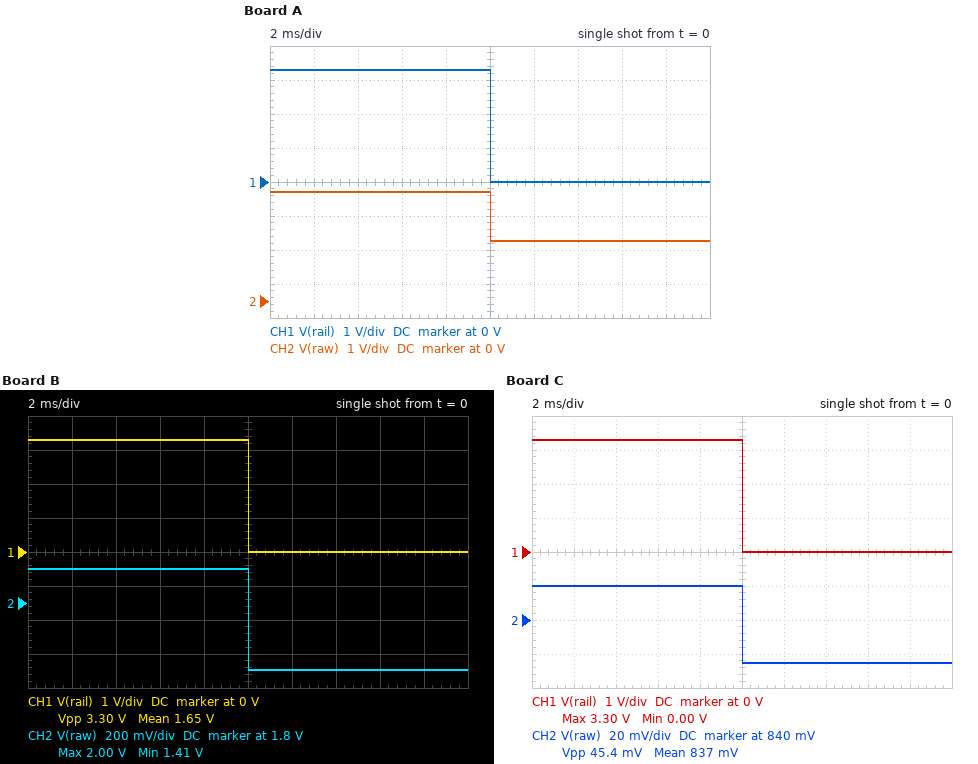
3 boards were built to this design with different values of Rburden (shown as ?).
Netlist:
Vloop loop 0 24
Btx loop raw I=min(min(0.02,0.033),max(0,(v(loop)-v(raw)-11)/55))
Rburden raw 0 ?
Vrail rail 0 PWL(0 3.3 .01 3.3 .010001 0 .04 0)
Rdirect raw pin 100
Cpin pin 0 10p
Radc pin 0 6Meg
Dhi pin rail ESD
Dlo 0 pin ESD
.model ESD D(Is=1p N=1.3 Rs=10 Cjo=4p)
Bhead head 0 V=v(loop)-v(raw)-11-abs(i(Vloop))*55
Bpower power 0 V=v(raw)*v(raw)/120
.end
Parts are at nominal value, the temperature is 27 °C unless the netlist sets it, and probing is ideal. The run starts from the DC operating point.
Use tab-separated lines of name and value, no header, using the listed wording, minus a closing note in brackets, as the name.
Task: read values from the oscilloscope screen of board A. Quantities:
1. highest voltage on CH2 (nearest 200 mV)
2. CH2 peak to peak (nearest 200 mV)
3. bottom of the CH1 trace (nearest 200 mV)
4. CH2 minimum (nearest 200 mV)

highest voltage on CH2	3.2 V
CH2 peak to peak	1.4 V
bottom of the CH1 trace	0 V
CH2 minimum	1.8 V
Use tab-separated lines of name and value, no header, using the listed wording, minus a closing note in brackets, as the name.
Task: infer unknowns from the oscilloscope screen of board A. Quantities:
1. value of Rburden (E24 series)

value of Rburden	160 Ω
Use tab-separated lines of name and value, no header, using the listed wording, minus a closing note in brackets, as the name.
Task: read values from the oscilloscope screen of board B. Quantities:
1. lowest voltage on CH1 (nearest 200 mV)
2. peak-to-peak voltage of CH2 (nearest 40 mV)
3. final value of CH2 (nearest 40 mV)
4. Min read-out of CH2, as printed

lowest voltage on CH1	0 V
peak-to-peak voltage of CH2	600 mV
final value of CH2	1.40 V
Min read-out of CH2, as printed	1.41 V
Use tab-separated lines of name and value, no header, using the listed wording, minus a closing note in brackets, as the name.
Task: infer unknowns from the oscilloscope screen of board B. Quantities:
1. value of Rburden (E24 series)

value of Rburden	100 Ω
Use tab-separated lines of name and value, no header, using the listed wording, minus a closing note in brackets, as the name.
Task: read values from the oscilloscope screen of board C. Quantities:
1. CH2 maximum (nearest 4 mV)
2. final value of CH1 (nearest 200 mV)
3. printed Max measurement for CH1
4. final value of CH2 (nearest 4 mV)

CH2 maximum	860 mV
final value of CH1	0 V
printed Max measurement for CH1	3.30 V
final value of CH2	816 mV
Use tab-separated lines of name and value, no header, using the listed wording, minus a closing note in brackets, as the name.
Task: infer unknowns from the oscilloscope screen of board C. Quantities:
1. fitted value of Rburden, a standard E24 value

fitted value of Rburden, a standard E24 value	43 Ω
